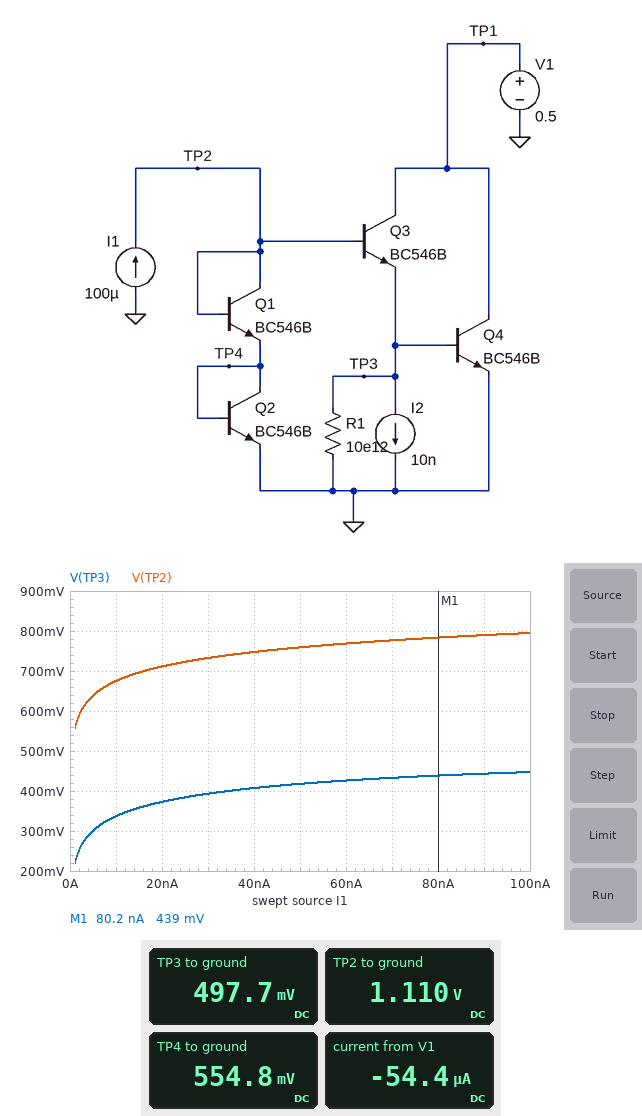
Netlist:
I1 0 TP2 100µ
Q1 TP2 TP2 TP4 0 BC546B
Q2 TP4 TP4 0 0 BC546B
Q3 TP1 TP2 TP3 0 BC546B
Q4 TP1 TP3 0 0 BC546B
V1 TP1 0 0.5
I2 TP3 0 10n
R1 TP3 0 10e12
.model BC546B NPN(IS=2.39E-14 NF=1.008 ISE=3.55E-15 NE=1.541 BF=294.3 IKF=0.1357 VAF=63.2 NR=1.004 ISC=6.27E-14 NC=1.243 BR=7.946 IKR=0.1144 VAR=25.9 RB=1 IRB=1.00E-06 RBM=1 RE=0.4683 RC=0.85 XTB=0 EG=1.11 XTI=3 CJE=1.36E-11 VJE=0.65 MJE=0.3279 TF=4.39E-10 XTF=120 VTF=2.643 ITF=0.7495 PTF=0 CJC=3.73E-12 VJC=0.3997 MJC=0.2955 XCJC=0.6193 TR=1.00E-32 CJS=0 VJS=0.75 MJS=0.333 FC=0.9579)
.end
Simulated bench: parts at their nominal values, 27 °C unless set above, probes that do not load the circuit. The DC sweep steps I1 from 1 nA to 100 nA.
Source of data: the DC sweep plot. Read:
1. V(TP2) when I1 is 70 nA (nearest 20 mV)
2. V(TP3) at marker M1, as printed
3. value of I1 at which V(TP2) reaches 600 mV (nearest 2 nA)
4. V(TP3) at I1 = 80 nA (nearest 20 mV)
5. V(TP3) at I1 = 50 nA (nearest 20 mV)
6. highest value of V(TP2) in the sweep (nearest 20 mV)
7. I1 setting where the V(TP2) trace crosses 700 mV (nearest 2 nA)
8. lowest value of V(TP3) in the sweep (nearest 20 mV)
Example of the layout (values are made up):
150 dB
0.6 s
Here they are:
780 mV
439 mV
2 nA
440 mV
420 mV
800 mV
16 nA
220 mV
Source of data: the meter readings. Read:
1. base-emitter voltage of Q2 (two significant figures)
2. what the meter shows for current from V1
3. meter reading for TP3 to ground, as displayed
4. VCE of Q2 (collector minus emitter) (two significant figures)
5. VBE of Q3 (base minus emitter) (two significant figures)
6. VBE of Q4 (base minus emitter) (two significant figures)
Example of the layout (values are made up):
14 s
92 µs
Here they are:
550 mV
-54.4 µA
497.7 mV
550 mV
610 mV
500 mV
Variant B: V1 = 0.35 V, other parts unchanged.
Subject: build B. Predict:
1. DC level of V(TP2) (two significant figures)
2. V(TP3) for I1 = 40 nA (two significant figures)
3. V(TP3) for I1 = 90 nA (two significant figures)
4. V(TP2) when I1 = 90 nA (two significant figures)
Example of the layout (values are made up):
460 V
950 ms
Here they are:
970 mV
340 mV
350 mV
760 mV
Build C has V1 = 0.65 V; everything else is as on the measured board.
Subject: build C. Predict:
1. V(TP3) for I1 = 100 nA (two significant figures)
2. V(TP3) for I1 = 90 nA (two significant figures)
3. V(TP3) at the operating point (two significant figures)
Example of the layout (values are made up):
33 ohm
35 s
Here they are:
450 mV
450 mV
640 mV
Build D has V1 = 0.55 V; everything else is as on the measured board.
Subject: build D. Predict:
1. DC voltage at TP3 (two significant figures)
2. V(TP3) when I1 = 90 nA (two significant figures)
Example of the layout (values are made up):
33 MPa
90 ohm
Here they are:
550 mV
450 mV
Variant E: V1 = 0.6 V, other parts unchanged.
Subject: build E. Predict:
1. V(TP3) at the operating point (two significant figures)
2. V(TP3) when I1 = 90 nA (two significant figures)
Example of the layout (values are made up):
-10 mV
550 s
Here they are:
600 mV
450 mV
